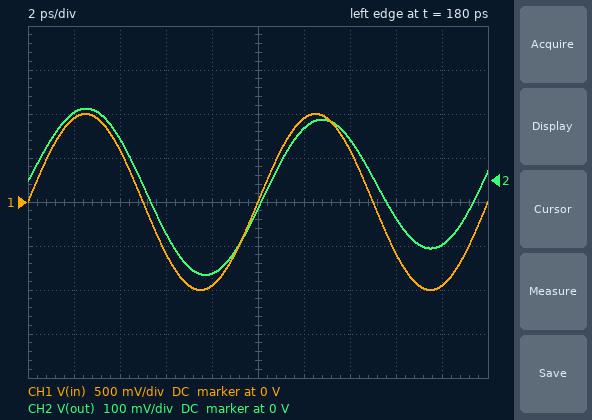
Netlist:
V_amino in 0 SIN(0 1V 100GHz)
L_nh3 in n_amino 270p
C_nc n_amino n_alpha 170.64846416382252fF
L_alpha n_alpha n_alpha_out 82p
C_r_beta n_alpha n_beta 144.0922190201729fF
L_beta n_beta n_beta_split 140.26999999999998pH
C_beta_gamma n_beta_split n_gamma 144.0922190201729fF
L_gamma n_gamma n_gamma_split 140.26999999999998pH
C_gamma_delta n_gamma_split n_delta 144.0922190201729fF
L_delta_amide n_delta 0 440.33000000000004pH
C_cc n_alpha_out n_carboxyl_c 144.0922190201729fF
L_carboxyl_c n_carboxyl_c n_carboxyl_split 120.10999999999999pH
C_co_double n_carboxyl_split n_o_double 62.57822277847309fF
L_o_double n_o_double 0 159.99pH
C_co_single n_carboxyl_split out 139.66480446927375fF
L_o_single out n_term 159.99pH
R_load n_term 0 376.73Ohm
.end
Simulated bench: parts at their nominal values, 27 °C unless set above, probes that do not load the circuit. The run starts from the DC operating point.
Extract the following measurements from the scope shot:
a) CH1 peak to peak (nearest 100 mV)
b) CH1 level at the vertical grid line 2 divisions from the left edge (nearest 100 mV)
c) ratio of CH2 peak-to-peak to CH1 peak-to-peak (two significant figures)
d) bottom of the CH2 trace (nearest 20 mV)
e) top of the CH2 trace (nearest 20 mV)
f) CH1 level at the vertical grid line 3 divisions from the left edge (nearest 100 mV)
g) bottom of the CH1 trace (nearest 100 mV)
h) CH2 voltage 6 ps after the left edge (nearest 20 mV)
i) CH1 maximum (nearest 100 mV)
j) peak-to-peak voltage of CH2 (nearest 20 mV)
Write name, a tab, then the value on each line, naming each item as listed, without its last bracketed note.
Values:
CH1 peak to peak	2.0 V
CH1 level at the vertical grid line 2 divisions from the left edge	600 mV
ratio of CH2 peak-to-peak to CH1 peak-to-peak	0.19
bottom of the CH2 trace	-220 mV
top of the CH2 trace	160 mV
CH1 level at the vertical grid line 3 divisions from the left edge	-600 mV
bottom of the CH1 trace	-1.0 V
CH2 voltage 6 ps after the left edge	-120 mV
CH1 maximum	1.0 V
peak-to-peak voltage of CH2	380 mV
